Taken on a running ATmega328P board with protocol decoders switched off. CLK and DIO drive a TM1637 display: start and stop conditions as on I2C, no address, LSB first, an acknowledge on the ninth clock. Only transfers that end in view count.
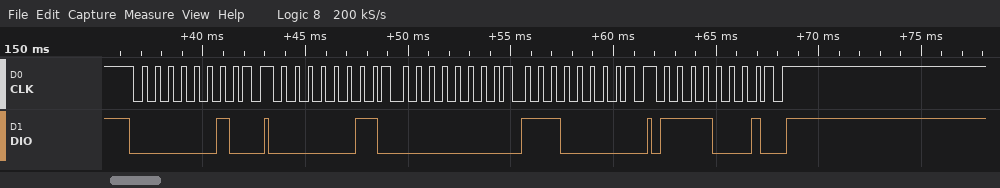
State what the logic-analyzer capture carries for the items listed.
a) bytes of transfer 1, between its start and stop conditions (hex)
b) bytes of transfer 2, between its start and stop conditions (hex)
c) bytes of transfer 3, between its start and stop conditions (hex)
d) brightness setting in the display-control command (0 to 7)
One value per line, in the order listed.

40
C0 00 07
8F
7
